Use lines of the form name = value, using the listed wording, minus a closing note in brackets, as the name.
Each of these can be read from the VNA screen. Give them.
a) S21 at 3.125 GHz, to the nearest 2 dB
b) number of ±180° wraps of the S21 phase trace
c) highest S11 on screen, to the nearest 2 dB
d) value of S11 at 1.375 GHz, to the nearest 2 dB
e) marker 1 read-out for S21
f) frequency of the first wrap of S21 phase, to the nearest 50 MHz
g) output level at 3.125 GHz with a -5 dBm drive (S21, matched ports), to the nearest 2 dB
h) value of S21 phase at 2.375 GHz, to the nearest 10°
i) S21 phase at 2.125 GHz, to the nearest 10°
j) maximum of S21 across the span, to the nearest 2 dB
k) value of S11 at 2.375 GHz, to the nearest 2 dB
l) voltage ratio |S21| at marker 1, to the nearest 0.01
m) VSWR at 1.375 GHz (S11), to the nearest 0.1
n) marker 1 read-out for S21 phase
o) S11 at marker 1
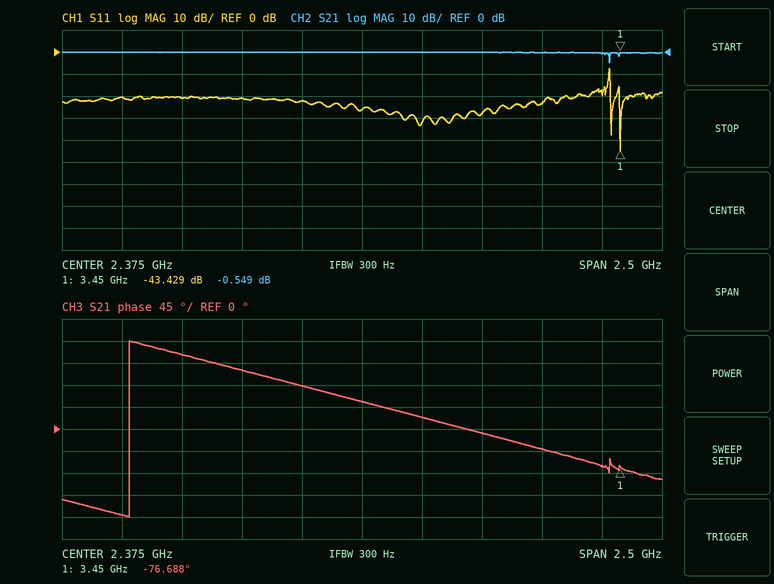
S21 at 3.125 GHz, to the nearest 2 dB = 0 dB
number of ±180° wraps of the S21 phase trace = 1
highest S11 on screen, to the nearest 2 dB = -8 dB
value of S11 at 1.375 GHz, to the nearest 2 dB = -20 dB
marker 1 read-out for S21 = -0.549 dB
frequency of the first wrap of S21 phase, to the nearest 50 MHz = 1.40 GHz
output level at 3.125 GHz with a -5 dBm drive (S21, matched ports), to the nearest 2 dB = -6 dBm
value of S21 phase at 2.375 GHz, to the nearest 10° = 60°
S21 phase at 2.125 GHz, to the nearest 10° = 90°
maximum of S21 across the span, to the nearest 2 dB = 0 dB
value of S11 at 2.375 GHz, to the nearest 2 dB = -26 dB
voltage ratio |S21| at marker 1, to the nearest 0.01 = 0.94
VSWR at 1.375 GHz (S11), to the nearest 0.1 = 1.2
marker 1 read-out for S21 phase = -76.688°
S11 at marker 1 = -43.429 dB
